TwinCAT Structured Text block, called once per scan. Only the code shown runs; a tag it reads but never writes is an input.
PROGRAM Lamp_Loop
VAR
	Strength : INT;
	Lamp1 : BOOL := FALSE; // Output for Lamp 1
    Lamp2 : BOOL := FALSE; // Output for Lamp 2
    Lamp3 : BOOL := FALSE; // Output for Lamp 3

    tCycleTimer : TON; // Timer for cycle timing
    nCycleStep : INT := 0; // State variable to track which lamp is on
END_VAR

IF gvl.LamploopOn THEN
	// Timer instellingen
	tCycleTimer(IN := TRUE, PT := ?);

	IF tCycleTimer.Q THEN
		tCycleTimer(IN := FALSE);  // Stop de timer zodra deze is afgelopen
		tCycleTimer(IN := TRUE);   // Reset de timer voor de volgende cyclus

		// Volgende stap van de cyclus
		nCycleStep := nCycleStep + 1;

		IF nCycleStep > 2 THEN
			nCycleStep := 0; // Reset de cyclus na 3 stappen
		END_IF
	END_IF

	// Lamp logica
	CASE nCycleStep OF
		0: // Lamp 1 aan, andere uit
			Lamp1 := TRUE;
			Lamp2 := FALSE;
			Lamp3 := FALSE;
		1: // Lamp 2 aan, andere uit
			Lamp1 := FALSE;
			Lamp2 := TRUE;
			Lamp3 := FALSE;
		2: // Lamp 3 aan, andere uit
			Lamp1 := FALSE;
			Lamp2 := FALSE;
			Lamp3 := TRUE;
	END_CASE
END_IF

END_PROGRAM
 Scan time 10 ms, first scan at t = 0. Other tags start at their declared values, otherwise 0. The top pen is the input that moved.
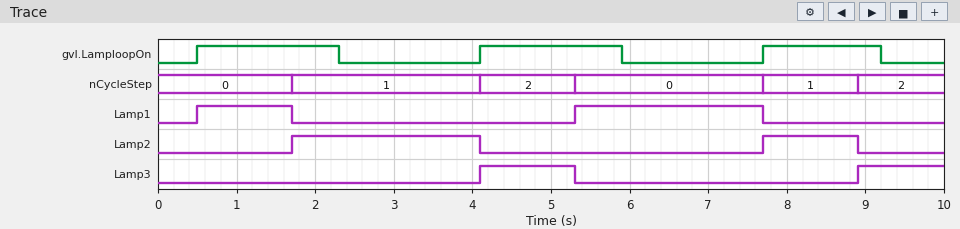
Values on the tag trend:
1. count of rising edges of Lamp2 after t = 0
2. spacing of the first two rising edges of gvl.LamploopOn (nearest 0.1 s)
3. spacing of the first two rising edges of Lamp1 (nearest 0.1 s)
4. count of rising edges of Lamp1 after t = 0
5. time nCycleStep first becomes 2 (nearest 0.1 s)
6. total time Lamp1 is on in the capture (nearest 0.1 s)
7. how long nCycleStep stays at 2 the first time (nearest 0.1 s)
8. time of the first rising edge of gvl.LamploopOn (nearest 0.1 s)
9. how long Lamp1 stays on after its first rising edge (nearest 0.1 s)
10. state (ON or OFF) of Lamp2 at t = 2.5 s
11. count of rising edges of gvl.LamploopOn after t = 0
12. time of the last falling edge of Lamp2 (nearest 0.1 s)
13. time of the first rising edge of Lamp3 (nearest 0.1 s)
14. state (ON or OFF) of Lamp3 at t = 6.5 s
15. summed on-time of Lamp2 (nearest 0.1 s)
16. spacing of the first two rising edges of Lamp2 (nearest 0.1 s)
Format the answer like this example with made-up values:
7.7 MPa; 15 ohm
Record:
2; 3.6 s; 4.8 s; 2; 4.1 s; 3.6 s; 1.2 s; 0.5 s; 1.2 s; ON; 3; 8.9 s; 4.1 s; OFF; 3.6 s; 6.0 s
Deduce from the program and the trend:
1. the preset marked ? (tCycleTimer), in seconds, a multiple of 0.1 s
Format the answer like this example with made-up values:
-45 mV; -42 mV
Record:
1.2 s
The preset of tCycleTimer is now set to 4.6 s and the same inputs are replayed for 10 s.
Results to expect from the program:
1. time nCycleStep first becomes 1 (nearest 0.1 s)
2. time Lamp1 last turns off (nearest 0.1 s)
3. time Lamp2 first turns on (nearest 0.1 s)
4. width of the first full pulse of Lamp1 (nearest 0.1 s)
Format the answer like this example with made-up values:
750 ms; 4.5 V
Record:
5.1 s; 5.1 s; 5.1 s; 4.6 s
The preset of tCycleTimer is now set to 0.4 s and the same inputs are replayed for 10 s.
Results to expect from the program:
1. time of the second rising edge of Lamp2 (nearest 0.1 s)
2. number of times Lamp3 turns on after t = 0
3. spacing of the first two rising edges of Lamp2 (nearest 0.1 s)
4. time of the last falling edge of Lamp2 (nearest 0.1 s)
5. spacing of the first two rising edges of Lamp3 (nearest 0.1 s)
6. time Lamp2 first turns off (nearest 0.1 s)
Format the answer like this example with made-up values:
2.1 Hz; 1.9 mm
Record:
2.1 s; 4; 1.2 s; 8.1 s; 2.8 s; 1.3 s
